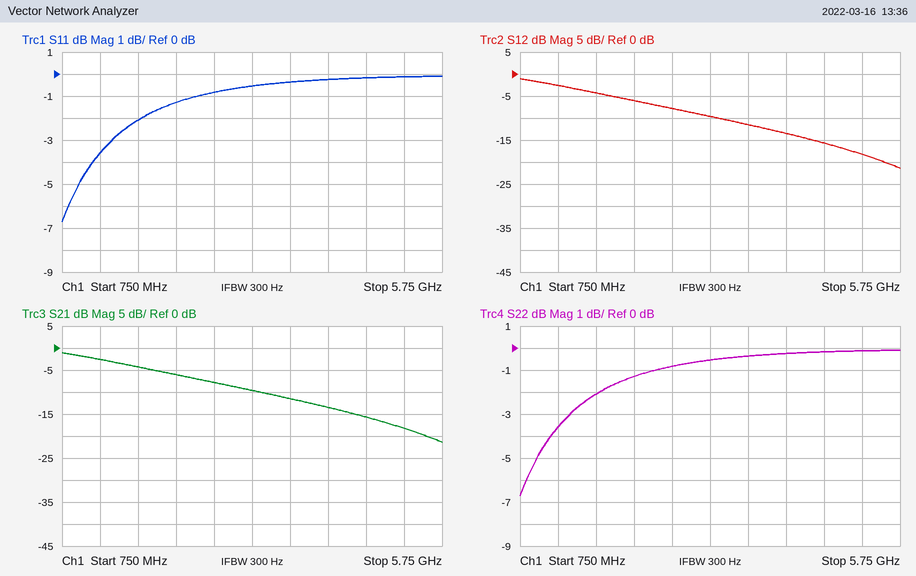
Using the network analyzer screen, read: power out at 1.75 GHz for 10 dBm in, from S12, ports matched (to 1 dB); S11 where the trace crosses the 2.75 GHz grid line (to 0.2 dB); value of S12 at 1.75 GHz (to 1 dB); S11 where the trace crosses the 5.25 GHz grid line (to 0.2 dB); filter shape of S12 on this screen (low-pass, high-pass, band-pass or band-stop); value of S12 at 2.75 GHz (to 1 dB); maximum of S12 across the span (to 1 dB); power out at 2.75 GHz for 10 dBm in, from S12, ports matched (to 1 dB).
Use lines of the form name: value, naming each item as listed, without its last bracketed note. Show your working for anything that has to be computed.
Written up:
power out at 1.75 GHz for 10 dBm in, from S12, ports matched: 10 dBm + (-4 dB) = 6 dBm
S11 where the trace crosses the 2.75 GHz grid line: -0.8 dB
value of S12 at 1.75 GHz: -4 dB
S11 where the trace crosses the 5.25 GHz grid line: -0.2 dB
filter shape of S12 on this screen: low-pass
value of S12 at 2.75 GHz: -8 dB
maximum of S12 across the span: -1 dB
power out at 2.75 GHz for 10 dBm in, from S12, ports matched: 10 dBm + (-8 dB) = 2 dBm
